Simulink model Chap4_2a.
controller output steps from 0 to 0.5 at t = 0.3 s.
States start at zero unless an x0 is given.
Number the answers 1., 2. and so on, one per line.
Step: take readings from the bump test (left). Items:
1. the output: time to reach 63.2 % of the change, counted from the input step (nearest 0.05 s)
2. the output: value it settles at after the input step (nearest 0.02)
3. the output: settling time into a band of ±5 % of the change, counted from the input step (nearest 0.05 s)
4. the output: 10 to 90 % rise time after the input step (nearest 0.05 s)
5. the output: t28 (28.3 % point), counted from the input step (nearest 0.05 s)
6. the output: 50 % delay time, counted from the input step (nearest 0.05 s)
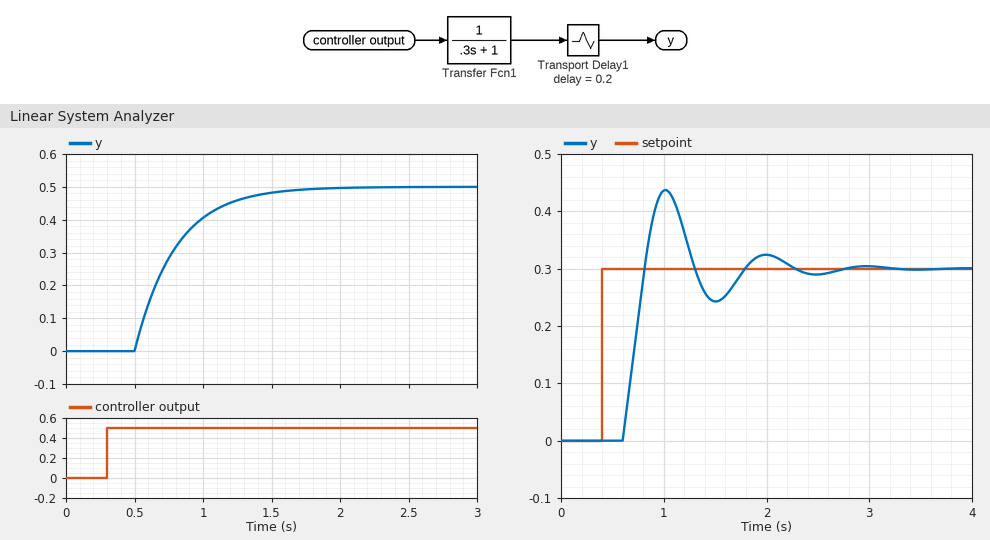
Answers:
1. 0.50 s
2. 0.50
3. 1.10 s
4. 0.65 s
5. 0.30 s
6. 0.40 s
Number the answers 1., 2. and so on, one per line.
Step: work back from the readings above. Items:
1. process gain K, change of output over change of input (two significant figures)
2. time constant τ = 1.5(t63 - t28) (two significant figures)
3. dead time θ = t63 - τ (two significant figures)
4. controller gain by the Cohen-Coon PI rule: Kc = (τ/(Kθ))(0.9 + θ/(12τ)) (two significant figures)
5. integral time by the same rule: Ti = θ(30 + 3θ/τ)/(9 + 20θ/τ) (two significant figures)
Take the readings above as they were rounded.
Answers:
1. 1.0
2. 0.30 s
3. 0.20 s
4. 1.4
5. 0.29 s
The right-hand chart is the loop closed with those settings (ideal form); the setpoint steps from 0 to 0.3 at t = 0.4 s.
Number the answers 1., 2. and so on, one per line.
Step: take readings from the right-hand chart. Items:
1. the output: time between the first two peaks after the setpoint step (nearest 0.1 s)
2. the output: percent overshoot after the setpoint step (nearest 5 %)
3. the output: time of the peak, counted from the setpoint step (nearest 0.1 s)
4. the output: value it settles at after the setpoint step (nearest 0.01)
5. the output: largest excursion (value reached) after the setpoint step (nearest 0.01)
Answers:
1. 1.0 s
2. 45 %
3. 0.6 s
4. 0.30
5. 0.44
